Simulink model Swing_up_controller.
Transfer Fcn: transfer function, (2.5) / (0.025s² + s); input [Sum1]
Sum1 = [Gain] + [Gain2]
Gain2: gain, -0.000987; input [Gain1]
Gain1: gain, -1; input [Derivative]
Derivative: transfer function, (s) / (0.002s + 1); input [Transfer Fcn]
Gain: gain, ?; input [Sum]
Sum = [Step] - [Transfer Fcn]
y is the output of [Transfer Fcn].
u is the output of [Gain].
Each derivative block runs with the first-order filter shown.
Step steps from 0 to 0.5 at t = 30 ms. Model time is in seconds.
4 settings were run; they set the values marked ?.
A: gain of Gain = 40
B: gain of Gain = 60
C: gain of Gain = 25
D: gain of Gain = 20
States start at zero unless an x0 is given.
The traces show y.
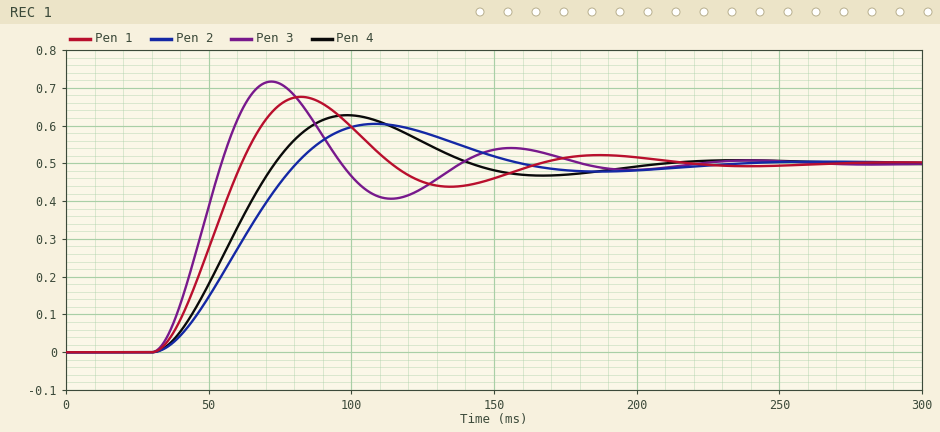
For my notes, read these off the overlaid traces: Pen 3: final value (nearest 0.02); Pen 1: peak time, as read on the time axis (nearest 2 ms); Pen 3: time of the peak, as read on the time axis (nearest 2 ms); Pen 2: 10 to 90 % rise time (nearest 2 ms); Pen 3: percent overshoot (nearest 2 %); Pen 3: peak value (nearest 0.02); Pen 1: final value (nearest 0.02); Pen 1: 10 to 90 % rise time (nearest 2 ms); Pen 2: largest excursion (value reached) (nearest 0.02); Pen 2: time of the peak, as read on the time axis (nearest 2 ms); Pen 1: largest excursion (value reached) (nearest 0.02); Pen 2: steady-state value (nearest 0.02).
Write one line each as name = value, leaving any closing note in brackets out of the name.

Pen 3: final value = 0.50
Pen 1: peak time, as read on the time axis = 82 ms
Pen 3: time of the peak, as read on the time axis = 72 ms
Pen 2: 10 to 90 % rise time = 34 ms
Pen 3: percent overshoot = 44 %
Pen 3: peak value = 0.72
Pen 1: final value = 0.50
Pen 1: 10 to 90 % rise time = 22 ms
Pen 2: largest excursion (value reached) = 0.60
Pen 2: time of the peak, as read on the time axis = 108 ms
Pen 1: largest excursion (value reached) = 0.68
Pen 2: steady-state value = 0.50
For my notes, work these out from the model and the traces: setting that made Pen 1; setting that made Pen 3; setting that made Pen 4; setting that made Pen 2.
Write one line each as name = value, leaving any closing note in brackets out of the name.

setting that made Pen 1 = A
setting that made Pen 3 = B
setting that made Pen 4 = C
setting that made Pen 2 = D
